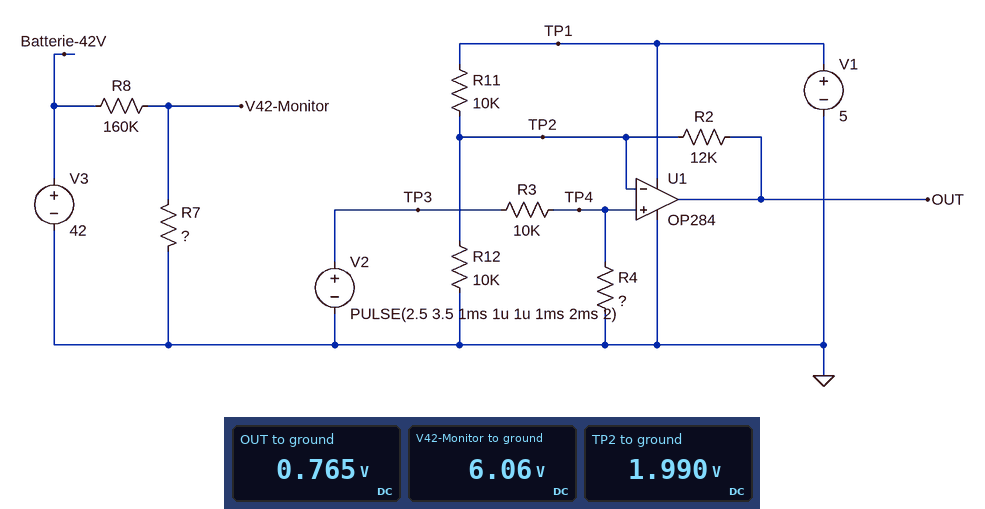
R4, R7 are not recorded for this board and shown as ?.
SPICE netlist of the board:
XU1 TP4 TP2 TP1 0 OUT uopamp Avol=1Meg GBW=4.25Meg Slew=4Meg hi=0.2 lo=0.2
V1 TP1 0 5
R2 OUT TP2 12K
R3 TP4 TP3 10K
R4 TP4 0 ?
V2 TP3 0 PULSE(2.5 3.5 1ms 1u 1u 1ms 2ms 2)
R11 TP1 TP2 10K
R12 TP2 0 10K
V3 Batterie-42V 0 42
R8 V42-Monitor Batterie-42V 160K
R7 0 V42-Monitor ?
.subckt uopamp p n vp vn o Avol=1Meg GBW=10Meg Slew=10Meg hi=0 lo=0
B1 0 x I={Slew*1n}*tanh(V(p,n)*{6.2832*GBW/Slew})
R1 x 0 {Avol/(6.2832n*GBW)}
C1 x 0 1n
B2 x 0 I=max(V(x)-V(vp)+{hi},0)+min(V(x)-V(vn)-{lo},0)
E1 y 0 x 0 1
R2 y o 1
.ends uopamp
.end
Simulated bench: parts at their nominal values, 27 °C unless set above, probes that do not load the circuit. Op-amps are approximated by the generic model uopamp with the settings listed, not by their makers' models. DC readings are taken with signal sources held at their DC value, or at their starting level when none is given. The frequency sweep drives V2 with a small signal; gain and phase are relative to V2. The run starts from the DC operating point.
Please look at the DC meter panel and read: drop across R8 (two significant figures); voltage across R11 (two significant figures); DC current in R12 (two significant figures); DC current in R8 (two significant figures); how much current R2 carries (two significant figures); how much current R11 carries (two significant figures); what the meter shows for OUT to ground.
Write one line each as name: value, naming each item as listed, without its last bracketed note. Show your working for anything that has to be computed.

drop across R8: 42 V - 6.06 V = 36 V
voltage across R11: 5 V - 1.99 V = 3.0 V
DC current in R12: (1.99 V) / 10 kΩ = 200 µA
DC current in R8: (42 V - 6.06 V) / 160 kΩ = 220 µA
how much current R2 carries: (1.99 V - 765 mV) / 12 kΩ = 100 µA
how much current R11 carries: (5 V - 1.99 V) / 10 kΩ = 300 µA
what the meter shows for OUT to ground: 0.765 V
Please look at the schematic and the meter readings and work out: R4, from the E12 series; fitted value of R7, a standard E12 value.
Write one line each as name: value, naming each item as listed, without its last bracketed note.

R4, from the E12 series: 39 kΩ
fitted value of R7, a standard E12 value: 27 kΩ
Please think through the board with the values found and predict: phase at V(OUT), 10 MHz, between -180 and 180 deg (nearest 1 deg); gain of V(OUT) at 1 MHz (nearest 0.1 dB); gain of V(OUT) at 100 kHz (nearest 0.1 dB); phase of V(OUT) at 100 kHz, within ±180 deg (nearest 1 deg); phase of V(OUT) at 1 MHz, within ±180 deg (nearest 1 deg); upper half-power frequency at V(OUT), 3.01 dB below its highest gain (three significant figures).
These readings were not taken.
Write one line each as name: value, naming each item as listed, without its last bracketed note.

phase at V(OUT), 10 MHz, between -180 and 180 deg: -83 deg
gain of V(OUT) at 1 MHz: 6.5 dB
gain of V(OUT) at 100 kHz: 8.6 dB
phase of V(OUT) at 100 kHz, within ±180 deg: -5 deg
phase of V(OUT) at 1 MHz, within ±180 deg: -39 deg
upper half-power frequency at V(OUT), 3.01 dB below its highest gain: 1.25 MHz
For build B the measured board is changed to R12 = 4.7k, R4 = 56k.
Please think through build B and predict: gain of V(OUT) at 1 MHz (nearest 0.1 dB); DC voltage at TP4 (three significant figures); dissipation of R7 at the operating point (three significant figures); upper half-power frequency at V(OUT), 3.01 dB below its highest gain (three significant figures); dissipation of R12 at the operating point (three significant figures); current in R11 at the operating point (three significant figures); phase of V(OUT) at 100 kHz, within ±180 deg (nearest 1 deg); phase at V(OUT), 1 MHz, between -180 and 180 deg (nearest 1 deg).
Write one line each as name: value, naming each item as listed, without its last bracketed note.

gain of V(OUT) at 1 MHz: 8.6 dB
DC voltage at TP4: 2.12 V
dissipation of R7 at the operating point: 1.36 mW
upper half-power frequency at V(OUT), 3.01 dB below its highest gain: 894 kHz
dissipation of R12 at the operating point: 957 µW
current in R11 at the operating point: 288 µA
phase of V(OUT) at 100 kHz, within ±180 deg: -6 deg
phase at V(OUT), 1 MHz, between -180 and 180 deg: -48 deg
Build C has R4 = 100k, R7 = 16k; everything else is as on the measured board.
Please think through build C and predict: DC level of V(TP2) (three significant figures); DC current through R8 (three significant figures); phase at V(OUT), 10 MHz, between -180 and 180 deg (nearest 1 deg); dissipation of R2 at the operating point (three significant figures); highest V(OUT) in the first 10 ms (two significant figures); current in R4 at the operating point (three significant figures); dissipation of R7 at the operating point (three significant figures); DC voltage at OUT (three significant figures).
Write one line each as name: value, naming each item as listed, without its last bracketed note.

DC level of V(TP2): 2.27 V
DC current through R8: 239 µA
phase at V(OUT), 10 MHz, between -180 and 180 deg: -83 deg
dissipation of R2 at the operating point: 24.8 µW
highest V(OUT) in the first 10 ms: 4.8 V
current in R4 at the operating point: 22.7 µA
dissipation of R7 at the operating point: 911 µW
DC voltage at OUT: 1.73 V
